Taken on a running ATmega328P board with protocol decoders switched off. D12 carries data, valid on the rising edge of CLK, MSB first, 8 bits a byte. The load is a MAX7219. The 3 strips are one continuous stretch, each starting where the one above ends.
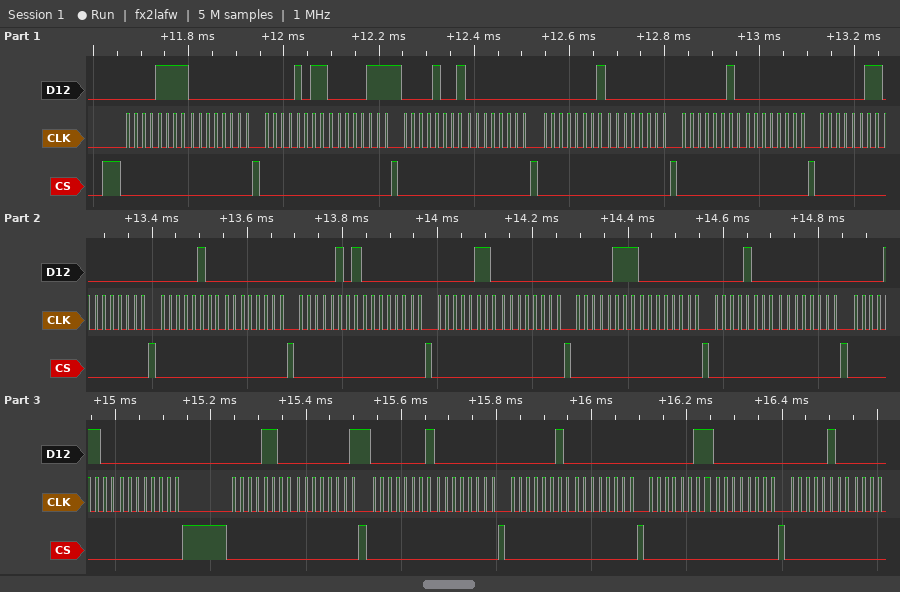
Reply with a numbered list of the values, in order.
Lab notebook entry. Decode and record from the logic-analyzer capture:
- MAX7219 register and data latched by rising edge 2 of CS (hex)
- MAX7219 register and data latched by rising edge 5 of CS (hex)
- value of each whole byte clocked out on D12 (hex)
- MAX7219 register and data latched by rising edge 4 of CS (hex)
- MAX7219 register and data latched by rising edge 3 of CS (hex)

1. register 0xF, data 0x00
2. register 0x1, data 0x00
3. 0x0F 0x00 0x0B 0x07 0x09 0x00 0x01 0x00 0x02 0x00 0x03 0x00 0x04 0x00 0x05 0x00 0x06 0x00 0x07 0x00 0x08 0x00 0x0C 0x00 0x0C 0x01 0x01 0x00 0x02 0x00 0x03 0x00 0x04
4. register 0x9, data 0x00
5. register 0xB, data 0x07
